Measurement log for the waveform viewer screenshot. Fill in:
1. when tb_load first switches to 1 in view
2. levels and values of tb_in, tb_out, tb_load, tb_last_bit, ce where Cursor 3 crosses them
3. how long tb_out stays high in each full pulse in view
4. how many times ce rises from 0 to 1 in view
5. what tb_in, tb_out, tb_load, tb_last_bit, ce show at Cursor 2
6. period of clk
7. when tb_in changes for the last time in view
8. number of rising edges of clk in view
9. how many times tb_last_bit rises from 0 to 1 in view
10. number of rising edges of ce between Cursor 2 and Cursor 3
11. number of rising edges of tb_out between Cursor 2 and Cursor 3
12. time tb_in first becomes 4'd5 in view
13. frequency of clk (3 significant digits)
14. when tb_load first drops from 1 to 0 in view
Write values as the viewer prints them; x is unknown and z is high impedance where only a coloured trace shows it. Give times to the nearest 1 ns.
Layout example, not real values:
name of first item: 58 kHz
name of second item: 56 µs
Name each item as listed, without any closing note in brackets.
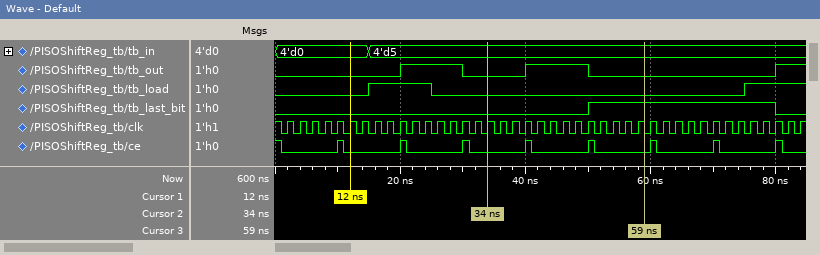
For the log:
when tb_load first switches to 1 in view: 15 ns
levels and values of tb_in, tb_out, tb_load, tb_last_bit, ce where Cursor 3 crosses them: tb_in=4'd5, tb_out=0, tb_load=0, tb_last_bit=1, ce=0
how long tb_out stays high in each full pulse in view: 10 ns, 10 ns
how many times ce rises from 0 to 1 in view: 8
what tb_in, tb_out, tb_load, tb_last_bit, ce show at Cursor 2: tb_in=4'd5, tb_out=0, tb_load=0, tb_last_bit=0, ce=0
period of clk: 2 ns
when tb_in changes for the last time in view: 15 ns
number of rising edges of clk in view: 42
how many times tb_last_bit rises from 0 to 1 in view: 1
number of rising edges of ce between Cursor 2 and Cursor 3: 2
number of rising edges of tb_out between Cursor 2 and Cursor 3: 1
time tb_in first becomes 4'd5 in view: 15 ns
frequency of clk: 500 MHz
when tb_load first drops from 1 to 0 in view: 25 ns
